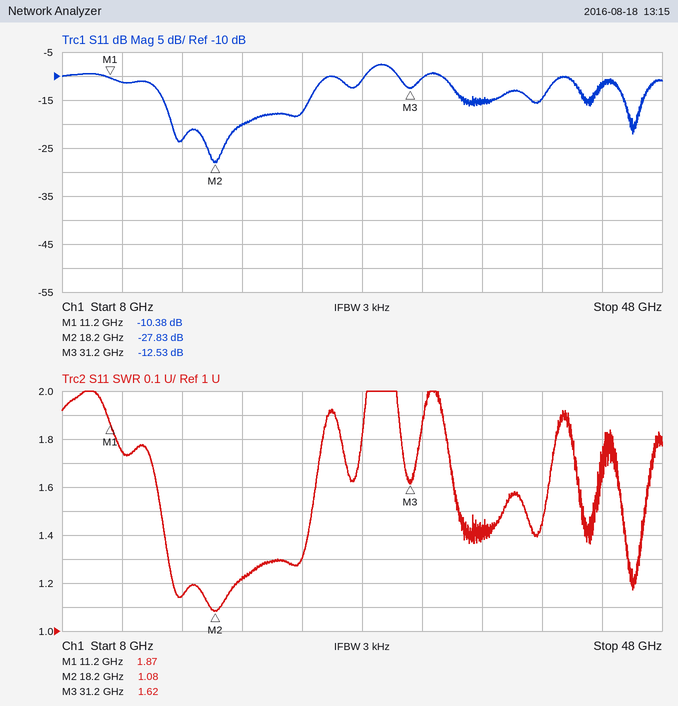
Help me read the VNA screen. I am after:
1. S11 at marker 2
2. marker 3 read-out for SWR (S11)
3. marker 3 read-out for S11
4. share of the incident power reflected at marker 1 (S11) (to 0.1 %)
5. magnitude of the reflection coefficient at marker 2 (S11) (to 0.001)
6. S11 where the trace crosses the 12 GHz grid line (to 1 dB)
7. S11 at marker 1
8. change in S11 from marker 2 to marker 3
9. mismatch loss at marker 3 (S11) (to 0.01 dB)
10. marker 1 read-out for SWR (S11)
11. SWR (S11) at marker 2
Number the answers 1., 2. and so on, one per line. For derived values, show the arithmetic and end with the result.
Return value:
1. -27.83 dB
2. 1.62
3. -12.53 dB
4. 10^(-10.38/10) ≈ 9.2 %
5. 10^(-27.83/20) ≈ 0.041
6. -11 dB
7. -10.38 dB
8. -12.53 − (-27.83) = 15.30 dB
9. −10 log10(1 − 10^(-12.53/10)) ≈ 0.25 dB
10. 1.87
11. 1.08
